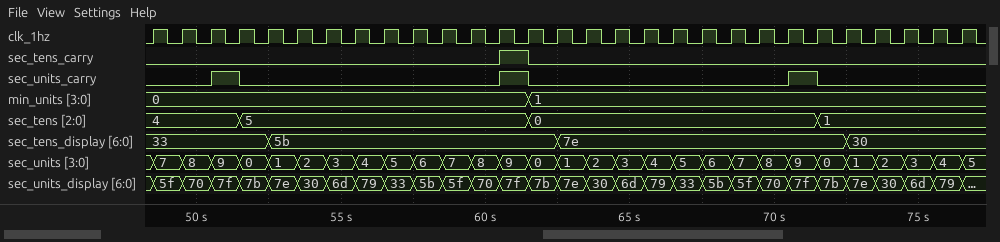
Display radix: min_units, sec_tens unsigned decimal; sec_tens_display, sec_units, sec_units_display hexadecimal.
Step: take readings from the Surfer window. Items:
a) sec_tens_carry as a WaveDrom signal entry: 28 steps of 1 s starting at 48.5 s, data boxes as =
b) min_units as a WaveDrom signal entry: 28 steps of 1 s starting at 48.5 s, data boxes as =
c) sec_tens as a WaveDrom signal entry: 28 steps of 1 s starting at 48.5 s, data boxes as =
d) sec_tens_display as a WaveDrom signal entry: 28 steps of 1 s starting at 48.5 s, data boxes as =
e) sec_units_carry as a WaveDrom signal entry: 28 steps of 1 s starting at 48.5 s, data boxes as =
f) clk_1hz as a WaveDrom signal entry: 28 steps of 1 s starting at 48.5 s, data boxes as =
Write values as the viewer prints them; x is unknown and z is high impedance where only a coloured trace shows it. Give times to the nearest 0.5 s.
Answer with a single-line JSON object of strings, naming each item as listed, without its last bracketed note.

{"sec_tens_carry as a WaveDrom signal entry: 28 steps of 1 s starting at 48.5 s, data boxes as =": "{name: 'sec_tens_carry', wave: '0...........10..............'}", "min_units as a WaveDrom signal entry: 28 steps of 1 s starting at 48.5 s, data boxes as =": "{name: 'min_units', wave: '=............=..............', data: '0 1'}", "sec_tens as a WaveDrom signal entry: 28 steps of 1 s starting at 48.5 s, data boxes as =": "{name: 'sec_tens', wave: '=..=.........=.........=....', data: '4 5 0 1'}", "sec_tens_display as a WaveDrom signal entry: 28 steps of 1 s starting at 48.5 s, data boxes as =": "{name: 'sec_tens_display', wave: '=...=.........=.........=...', data: '33 5b 7e 30'}", "sec_units_carry as a WaveDrom signal entry: 28 steps of 1 s starting at 48.5 s, data boxes as =": "{name: 'sec_units_carry', wave: '0.10........10........10....'}", "clk_1hz as a WaveDrom signal entry: 28 steps of 1 s starting at 48.5 s, data boxes as =": "{name: 'clk_1hz', wave: 'p...........................'}"}
